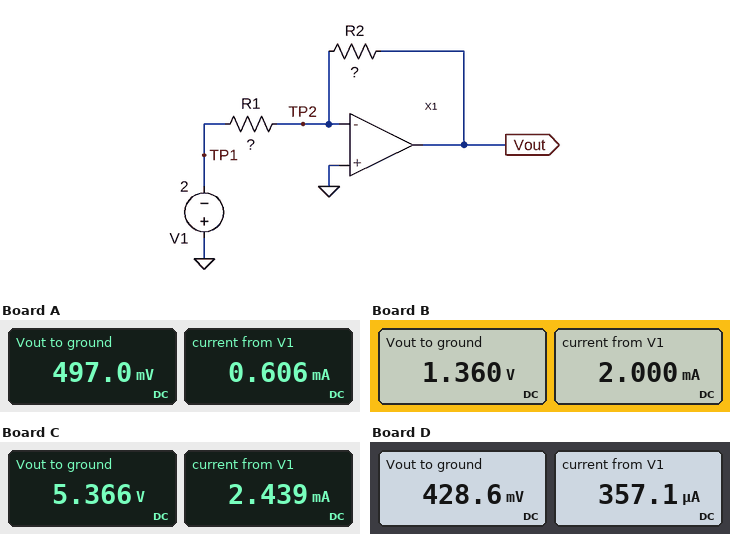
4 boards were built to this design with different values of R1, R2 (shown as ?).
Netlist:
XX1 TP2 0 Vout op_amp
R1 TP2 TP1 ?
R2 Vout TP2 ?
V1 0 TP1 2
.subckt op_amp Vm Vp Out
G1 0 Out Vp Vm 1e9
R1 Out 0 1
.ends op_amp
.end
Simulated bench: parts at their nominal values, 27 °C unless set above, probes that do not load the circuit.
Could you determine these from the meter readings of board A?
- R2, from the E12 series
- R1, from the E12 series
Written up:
820 Ω
3.3 kΩ
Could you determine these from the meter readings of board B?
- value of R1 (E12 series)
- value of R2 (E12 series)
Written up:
1 kΩ
680 Ω
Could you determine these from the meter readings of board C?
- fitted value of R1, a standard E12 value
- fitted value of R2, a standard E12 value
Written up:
820 Ω
2.2 kΩ
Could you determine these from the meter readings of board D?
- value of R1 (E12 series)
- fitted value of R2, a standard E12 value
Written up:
5.6 kΩ
1.2 kΩ
